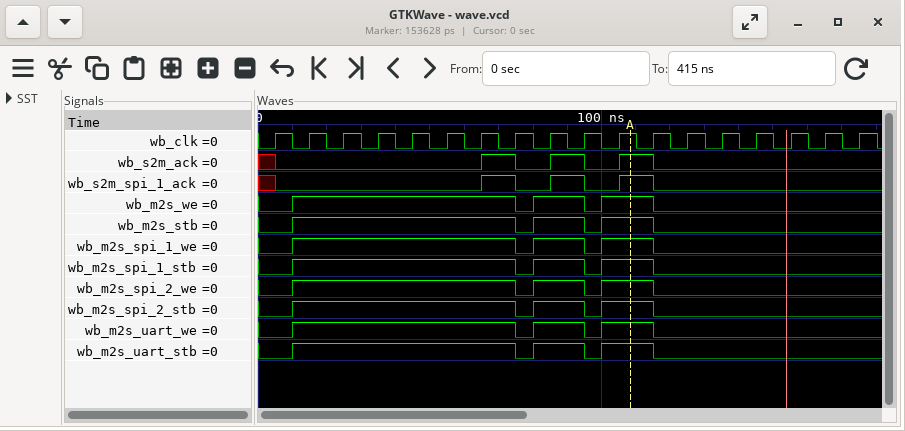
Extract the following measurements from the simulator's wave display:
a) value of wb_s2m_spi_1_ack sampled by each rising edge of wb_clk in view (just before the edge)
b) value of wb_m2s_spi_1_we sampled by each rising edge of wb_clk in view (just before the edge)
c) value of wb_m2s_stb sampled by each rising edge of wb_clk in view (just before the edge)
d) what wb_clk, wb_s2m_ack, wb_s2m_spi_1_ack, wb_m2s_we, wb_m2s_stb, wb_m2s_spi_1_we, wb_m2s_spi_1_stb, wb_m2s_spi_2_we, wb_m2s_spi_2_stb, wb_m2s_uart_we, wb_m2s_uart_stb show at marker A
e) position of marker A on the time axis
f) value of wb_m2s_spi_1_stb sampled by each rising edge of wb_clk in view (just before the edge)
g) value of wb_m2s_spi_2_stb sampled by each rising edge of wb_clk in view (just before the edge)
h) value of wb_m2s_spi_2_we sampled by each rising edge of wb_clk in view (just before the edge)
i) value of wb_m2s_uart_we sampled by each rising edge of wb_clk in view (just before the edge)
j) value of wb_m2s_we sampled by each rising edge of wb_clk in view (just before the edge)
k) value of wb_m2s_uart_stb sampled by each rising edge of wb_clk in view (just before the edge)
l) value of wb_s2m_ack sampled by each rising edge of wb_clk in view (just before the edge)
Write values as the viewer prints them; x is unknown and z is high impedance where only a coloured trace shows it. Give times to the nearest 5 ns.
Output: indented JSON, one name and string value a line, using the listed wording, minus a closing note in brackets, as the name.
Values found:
{
  "value of wb_s2m_spi_1_ack sampled by each rising edge of wb_clk in view": "x 0 0 0 0 0 0 1 0 1 0 1 0 0 0 0 0 0",
  "value of wb_m2s_spi_1_we sampled by each rising edge of wb_clk in view": "0 1 1 1 1 1 1 1 1 1 1 1 0 0 0 0 0 0",
  "value of wb_m2s_stb sampled by each rising edge of wb_clk in view": "0 1 1 1 1 1 1 1 1 1 1 1 0 0 0 0 0 0",
  "what wb_clk, wb_s2m_ack, wb_s2m_spi_1_ack, wb_m2s_we, wb_m2s_stb, wb_m2s_spi_1_we, wb_m2s_spi_1_stb, wb_m2s_spi_2_we, wb_m2s_spi_2_stb, wb_m2s_uart_we, wb_m2s_uart_stb show at marker A": "wb_clk=1, wb_s2m_ack=1, wb_s2m_spi_1_ack=1, wb_m2s_we=1, wb_m2s_stb=1, wb_m2s_spi_1_we=1, wb_m2s_spi_1_stb=1, wb_m2s_spi_2_we=1, wb_m2s_spi_2_stb=1, wb_m2s_uart_we=1, wb_m2s_uart_stb=1",
  "position of marker A on the time axis": "110 ns",
  "value of wb_m2s_spi_1_stb sampled by each rising edge of wb_clk in view": "0 1 1 1 1 1 1 1 1 1 1 1 0 0 0 0 0 0",
  "value of wb_m2s_spi_2_stb sampled by each rising edge of wb_clk in view": "0 1 1 1 1 1 1 1 1 1 1 1 0 0 0 0 0 0",
  "value of wb_m2s_spi_2_we sampled by each rising edge of wb_clk in view": "0 1 1 1 1 1 1 1 1 1 1 1 0 0 0 0 0 0",
  "value of wb_m2s_uart_we sampled by each rising edge of wb_clk in view": "0 1 1 1 1 1 1 1 1 1 1 1 0 0 0 0 0 0",
  "value of wb_m2s_we sampled by each rising edge of wb_clk in view": "0 1 1 1 1 1 1 1 1 1 1 1 0 0 0 0 0 0",
  "value of wb_m2s_uart_stb sampled by each rising edge of wb_clk in view": "0 1 1 1 1 1 1 1 1 1 1 1 0 0 0 0 0 0",
  "value of wb_s2m_ack sampled by each rising edge of wb_clk in view": "x 0 0 0 0 0 0 1 0 1 0 1 0 0 0 0 0 0"
}
